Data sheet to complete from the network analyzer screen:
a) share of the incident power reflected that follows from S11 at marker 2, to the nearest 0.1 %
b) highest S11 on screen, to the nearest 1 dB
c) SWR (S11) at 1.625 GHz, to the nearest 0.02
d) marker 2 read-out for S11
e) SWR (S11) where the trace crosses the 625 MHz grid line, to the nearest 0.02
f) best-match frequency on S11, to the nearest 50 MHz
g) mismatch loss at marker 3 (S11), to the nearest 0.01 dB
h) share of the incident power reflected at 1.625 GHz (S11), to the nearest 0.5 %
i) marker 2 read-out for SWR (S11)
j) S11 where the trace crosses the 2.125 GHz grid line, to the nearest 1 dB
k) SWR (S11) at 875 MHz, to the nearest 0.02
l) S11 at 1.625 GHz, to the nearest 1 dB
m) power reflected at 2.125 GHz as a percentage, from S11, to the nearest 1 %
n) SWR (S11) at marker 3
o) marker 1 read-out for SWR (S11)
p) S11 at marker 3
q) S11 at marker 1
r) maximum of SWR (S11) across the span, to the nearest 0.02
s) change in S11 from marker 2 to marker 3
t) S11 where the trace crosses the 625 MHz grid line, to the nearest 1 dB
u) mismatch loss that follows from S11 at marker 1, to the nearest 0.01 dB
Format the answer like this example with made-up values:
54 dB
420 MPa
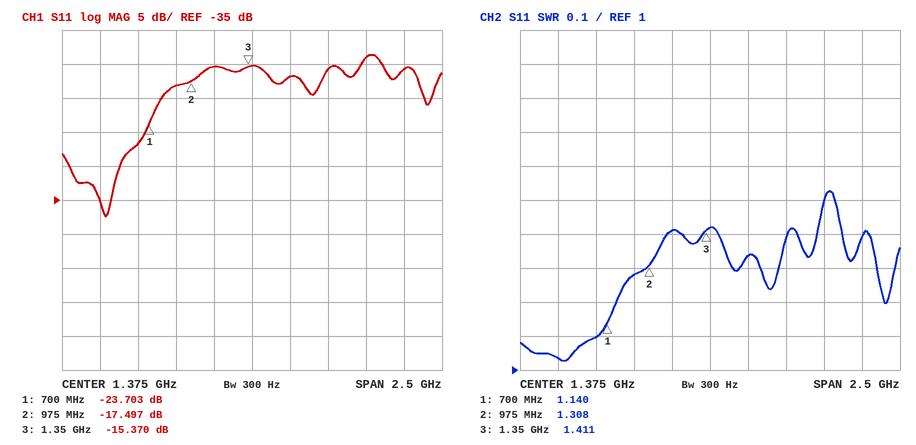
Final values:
1.8 %
-14 dB
1.34
-17.497 dB
1.10
400 MHz
0.13 dB
2.0 %
1.308
-14 dB
1.28
-17 dB
4 %
1.411
1.140
-15.370 dB
-23.703 dB
1.52
2.127 dB
-27 dB
0.02 dB
